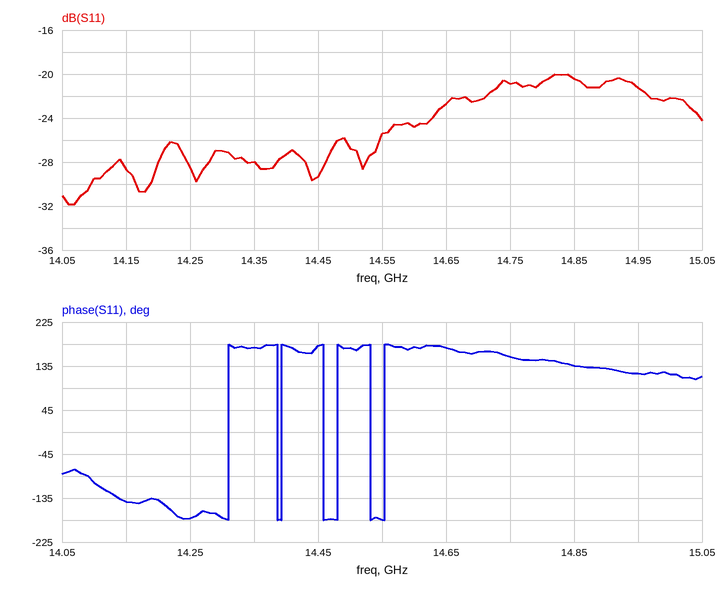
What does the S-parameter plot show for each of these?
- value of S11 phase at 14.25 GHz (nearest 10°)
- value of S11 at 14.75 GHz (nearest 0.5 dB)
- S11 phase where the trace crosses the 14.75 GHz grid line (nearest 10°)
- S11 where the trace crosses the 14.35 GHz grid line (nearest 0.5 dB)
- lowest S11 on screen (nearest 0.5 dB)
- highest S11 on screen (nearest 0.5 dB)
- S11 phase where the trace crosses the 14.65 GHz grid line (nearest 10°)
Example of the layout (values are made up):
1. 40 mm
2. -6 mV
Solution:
1. -180°
2. -21.0 dB
3. 150°
4. -28.0 dB
5. -32.0 dB
6. -20.0 dB
7. 170°
